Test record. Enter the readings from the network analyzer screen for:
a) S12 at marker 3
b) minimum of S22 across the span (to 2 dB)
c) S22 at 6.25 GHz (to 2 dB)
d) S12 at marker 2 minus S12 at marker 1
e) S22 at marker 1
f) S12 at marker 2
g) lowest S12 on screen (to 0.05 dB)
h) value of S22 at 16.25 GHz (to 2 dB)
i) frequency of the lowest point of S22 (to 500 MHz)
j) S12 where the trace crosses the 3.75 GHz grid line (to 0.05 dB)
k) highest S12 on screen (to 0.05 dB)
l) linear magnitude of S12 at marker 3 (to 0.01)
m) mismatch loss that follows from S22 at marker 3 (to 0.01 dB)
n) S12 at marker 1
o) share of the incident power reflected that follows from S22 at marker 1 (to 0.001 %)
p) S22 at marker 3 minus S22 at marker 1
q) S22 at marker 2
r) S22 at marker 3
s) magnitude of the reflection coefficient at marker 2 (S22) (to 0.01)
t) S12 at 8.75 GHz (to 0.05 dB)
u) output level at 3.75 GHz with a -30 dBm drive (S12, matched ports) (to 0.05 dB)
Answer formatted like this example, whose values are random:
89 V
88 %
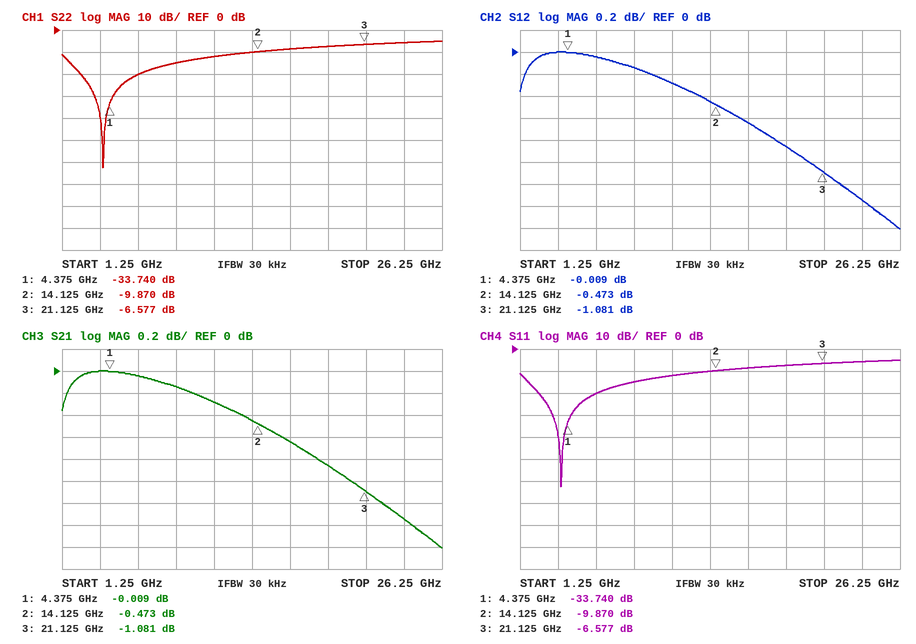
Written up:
-1.081 dB
-62 dB
-20 dB
-0.464 dB
-33.740 dB
-0.473 dB
-1.60 dB
-8 dB
4.0 GHz
0.00 dB
0.00 dB
0.88
1.08 dB
-0.009 dB
0.042 %
27.163 dB
-9.870 dB
-6.577 dB
0.32
-0.15 dB
-30.00 dBm
